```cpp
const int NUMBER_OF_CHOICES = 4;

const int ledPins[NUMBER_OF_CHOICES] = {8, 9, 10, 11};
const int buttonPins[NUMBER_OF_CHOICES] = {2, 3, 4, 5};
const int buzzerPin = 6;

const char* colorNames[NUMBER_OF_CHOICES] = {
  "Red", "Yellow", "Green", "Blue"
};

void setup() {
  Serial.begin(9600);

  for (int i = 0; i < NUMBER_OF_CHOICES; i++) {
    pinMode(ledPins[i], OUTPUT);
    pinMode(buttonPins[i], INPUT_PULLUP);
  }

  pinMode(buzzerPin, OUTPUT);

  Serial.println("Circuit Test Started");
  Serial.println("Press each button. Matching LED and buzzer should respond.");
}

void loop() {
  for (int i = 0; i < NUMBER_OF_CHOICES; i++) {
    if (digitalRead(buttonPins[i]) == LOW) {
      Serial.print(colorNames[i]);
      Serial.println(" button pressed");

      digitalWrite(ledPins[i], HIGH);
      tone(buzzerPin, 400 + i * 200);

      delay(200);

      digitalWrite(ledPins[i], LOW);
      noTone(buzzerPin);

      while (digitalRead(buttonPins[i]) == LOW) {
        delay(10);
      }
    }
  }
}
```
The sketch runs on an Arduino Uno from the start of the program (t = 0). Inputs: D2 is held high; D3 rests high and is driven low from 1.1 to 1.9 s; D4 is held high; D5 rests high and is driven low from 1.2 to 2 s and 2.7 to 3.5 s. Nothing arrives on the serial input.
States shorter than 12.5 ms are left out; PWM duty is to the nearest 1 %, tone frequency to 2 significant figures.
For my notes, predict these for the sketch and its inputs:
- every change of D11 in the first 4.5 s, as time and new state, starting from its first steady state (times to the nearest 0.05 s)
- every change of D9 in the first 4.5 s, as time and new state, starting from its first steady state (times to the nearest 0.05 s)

0 s low; 1.9 s high; 2.1 s low; 2.7 s high; 2.9 s low
0 s low; 1.1 s high; 1.3 s low
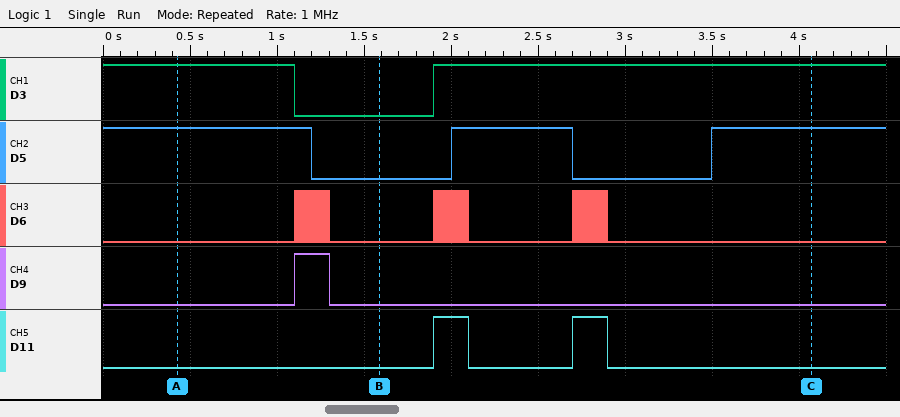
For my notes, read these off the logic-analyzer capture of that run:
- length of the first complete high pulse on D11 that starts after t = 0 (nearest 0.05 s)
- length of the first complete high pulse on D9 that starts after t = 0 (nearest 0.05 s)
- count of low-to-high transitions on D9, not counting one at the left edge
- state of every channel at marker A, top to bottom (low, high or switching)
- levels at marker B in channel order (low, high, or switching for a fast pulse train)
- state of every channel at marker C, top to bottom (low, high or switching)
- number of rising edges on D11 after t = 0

0.20 s
0.20 s
1
D3 high, D5 high, D6 low, D9 low, D11 low
D3 low, D5 low, D6 low, D9 low, D11 low
D3 high, D5 high, D6 low, D9 low, D11 low
2
